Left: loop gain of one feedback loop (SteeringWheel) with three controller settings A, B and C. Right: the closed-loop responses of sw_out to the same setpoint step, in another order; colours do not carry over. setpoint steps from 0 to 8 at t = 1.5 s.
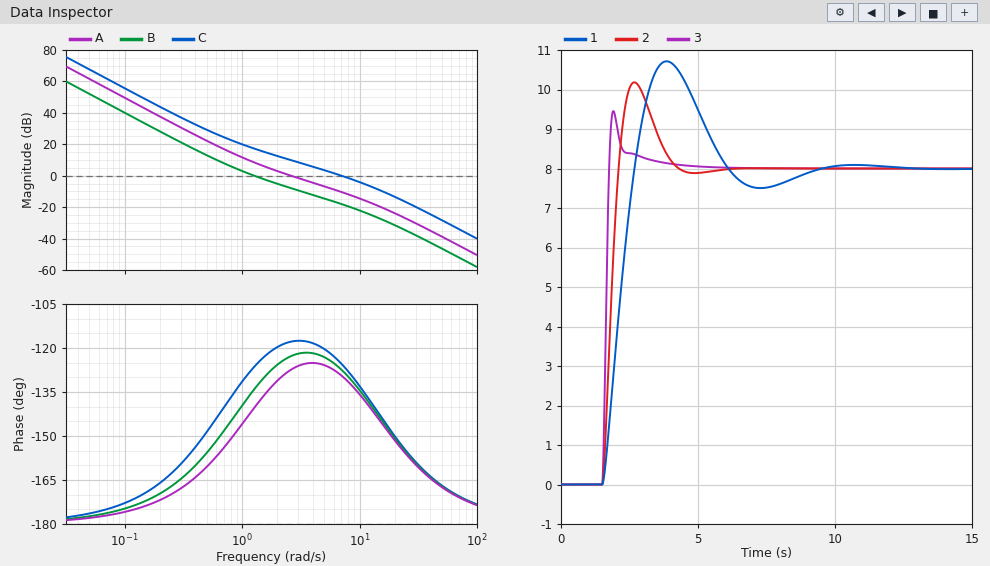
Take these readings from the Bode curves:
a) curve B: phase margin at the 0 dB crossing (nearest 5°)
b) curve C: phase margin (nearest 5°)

45°
55°
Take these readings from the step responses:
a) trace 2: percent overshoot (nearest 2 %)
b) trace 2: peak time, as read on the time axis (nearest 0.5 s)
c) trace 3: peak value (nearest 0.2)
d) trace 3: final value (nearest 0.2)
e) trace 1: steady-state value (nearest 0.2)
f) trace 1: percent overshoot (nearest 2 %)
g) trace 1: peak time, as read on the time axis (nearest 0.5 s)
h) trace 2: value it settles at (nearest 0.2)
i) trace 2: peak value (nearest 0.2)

28 %
2.5 s
9.4
8.0
8.0
34 %
4.0 s
8.0
10.2
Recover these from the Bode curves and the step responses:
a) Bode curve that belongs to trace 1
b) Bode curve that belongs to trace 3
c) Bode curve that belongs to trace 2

B
C
A
